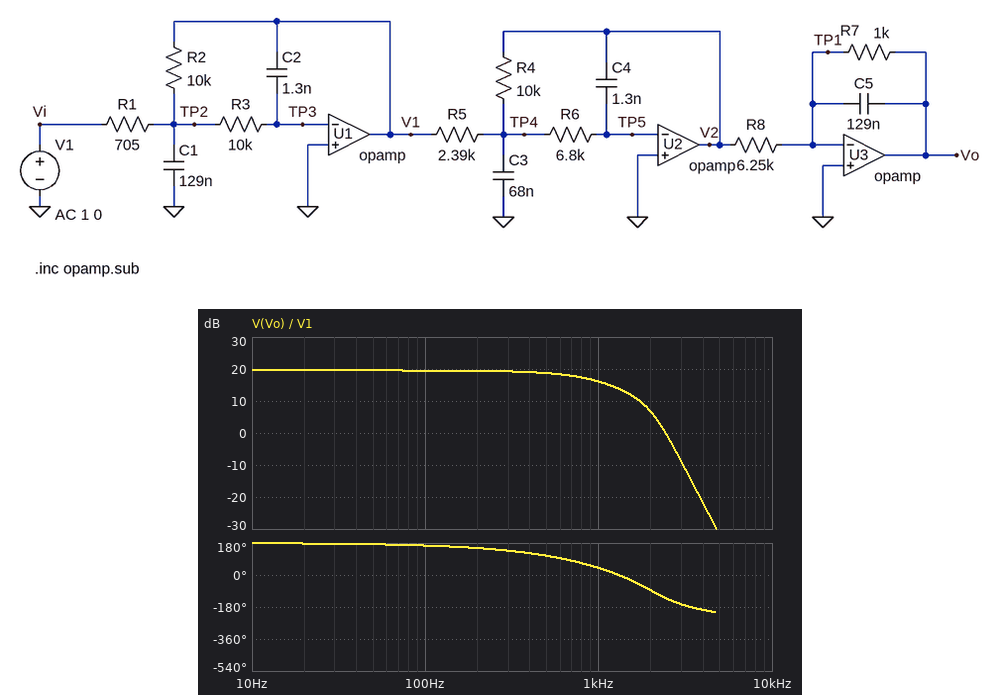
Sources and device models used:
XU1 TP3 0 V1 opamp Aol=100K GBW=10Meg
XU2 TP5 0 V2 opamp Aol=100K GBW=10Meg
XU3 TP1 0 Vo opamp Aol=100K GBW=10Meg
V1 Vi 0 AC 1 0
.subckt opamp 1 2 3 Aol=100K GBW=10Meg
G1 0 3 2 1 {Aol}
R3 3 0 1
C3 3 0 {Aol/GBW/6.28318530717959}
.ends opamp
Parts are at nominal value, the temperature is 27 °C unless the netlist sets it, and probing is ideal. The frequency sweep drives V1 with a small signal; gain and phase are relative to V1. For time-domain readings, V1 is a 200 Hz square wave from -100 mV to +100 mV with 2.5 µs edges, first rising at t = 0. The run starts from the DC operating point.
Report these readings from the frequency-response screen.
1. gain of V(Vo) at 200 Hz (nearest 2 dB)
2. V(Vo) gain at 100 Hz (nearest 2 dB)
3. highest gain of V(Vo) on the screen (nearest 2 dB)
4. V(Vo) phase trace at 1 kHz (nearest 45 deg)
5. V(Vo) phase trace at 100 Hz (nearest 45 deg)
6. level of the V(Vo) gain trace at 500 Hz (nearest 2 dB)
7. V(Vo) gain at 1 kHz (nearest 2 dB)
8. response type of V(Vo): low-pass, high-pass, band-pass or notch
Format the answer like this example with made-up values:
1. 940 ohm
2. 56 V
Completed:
1. 20 dB
2. 20 dB
3. 20 dB
4. 45 deg
5. 180 deg
6. 18 dB
7. 16 dB
8. low-pass
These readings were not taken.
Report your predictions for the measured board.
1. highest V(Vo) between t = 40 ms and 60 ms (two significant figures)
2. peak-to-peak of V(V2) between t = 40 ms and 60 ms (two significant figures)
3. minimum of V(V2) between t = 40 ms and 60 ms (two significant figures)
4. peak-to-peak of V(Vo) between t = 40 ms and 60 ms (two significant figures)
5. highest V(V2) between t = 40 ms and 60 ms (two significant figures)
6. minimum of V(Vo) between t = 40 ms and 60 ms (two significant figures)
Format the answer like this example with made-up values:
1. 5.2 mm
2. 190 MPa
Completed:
1. 960 mV
2. 13 V
3. -6.4 V
4. 1.9 V
5. 6.4 V
6. -960 mV
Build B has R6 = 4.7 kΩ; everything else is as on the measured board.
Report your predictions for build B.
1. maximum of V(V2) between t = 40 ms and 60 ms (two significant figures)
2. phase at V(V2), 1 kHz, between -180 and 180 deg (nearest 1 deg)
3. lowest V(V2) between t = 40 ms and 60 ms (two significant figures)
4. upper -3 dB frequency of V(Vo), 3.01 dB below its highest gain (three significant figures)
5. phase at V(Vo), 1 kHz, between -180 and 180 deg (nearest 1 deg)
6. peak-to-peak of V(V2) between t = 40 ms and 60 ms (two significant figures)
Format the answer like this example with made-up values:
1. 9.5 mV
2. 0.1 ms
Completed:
1. 6.1 V
2. -94 deg
3. -6.1 V
4. 887 Hz
5. 47 deg
6. 12 V
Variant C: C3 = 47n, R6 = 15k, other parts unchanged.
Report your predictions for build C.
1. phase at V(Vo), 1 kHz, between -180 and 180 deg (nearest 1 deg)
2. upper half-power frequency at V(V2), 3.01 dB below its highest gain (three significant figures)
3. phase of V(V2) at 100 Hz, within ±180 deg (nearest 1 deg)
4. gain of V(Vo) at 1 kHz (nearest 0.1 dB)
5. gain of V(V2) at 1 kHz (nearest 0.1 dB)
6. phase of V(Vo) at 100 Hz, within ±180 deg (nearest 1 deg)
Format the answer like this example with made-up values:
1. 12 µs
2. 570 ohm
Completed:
1. 17 deg
2. 1.09 kHz
3. -12 deg
4. 15.0 dB
5. 33.1 dB
6. 164 deg
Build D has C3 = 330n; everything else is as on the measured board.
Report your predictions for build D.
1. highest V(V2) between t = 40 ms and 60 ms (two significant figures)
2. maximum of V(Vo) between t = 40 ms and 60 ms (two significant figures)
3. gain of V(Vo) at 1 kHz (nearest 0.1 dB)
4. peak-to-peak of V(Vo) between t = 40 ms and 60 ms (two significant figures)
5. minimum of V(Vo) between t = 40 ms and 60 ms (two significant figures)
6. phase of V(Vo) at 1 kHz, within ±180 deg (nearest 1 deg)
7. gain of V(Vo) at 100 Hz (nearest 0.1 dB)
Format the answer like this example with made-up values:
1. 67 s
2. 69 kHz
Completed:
1. 11 V
2. 1.6 V
3. 22.6 dB
4. 3.2 V
5. -1.6 V
6. -47 deg
7. 19.6 dB
